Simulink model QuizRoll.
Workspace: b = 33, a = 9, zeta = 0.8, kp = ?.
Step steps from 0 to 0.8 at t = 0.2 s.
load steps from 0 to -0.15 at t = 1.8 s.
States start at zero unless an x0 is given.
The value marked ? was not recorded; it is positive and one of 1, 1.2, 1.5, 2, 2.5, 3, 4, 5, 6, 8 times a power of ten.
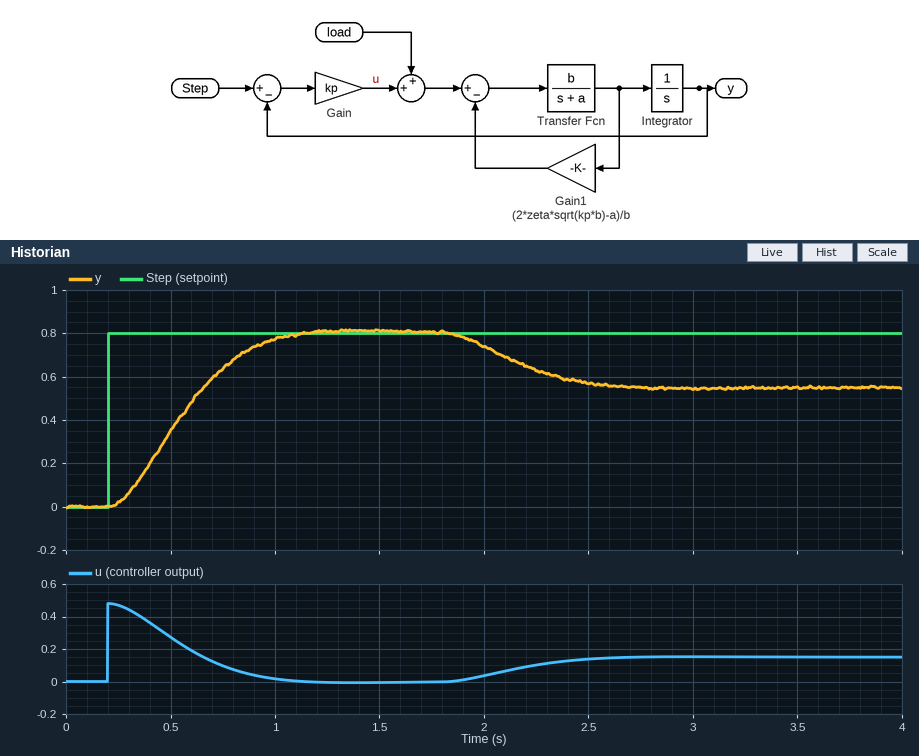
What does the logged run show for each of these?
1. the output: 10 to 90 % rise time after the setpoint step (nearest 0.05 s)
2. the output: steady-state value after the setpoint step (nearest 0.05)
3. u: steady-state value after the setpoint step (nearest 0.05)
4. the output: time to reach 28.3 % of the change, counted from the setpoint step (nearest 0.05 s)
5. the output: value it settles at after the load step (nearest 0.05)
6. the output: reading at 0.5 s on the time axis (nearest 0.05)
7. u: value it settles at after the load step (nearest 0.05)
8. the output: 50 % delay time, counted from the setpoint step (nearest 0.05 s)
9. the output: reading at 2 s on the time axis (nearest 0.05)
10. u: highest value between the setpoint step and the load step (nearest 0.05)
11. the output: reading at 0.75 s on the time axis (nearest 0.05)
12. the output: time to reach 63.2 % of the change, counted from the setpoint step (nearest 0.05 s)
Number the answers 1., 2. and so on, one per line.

1. 0.55 s
2. 0.80
3. 0.00
4. 0.20 s
5. 0.55
6. 0.35
7. 0.15
8. 0.35 s
9. 0.75
10. 0.50
11. 0.65
12. 0.40 s
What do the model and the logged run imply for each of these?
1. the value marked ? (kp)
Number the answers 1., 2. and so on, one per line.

1. 0.6
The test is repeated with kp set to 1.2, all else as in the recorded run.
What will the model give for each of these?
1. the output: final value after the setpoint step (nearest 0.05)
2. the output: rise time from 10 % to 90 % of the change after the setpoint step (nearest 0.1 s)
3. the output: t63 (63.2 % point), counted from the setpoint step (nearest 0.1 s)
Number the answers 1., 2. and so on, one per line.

1. 0.80
2. 0.4 s
3. 0.3 s
